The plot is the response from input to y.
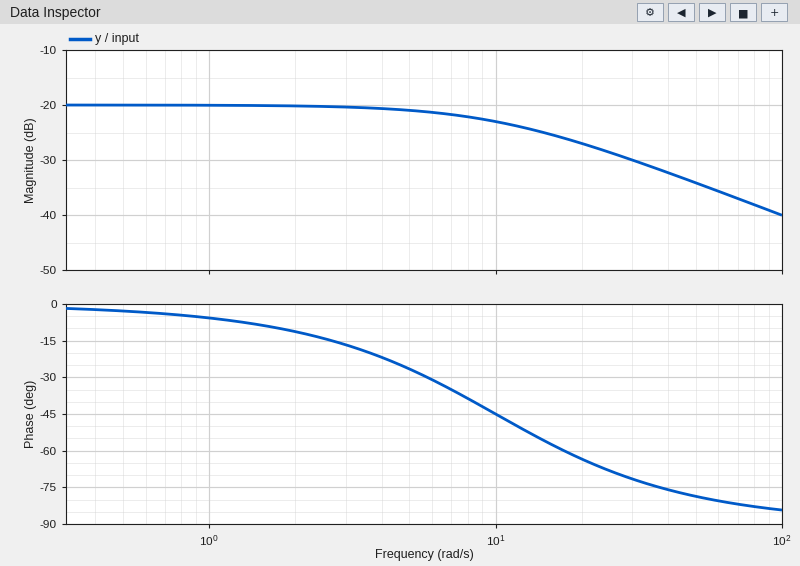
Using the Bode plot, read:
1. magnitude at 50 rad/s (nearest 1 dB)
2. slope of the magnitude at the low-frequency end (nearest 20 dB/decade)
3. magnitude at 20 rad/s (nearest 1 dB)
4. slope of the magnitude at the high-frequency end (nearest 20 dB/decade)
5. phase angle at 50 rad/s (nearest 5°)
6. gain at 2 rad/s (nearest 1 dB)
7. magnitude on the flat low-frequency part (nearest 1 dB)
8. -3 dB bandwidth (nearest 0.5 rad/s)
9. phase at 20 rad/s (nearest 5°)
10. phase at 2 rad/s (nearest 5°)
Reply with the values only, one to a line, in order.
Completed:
-34 dB
0 dB/decade
-27 dB
-20 dB/decade
-80°
-20 dB
-20 dB
10.0 rad/s
-65°
-10°
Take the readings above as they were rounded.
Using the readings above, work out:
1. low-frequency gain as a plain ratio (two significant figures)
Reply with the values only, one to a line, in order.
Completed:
0.10
